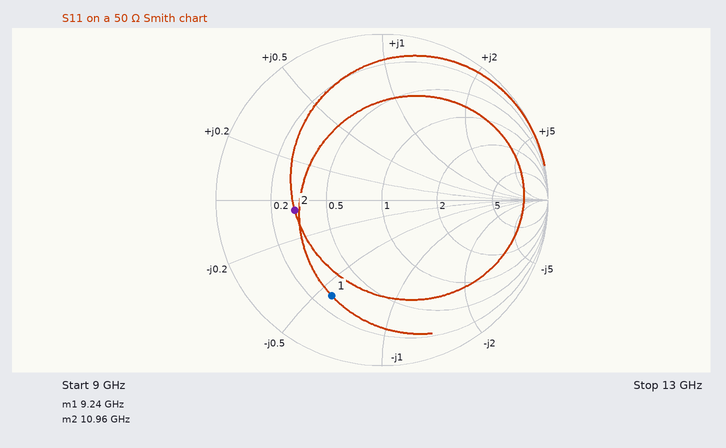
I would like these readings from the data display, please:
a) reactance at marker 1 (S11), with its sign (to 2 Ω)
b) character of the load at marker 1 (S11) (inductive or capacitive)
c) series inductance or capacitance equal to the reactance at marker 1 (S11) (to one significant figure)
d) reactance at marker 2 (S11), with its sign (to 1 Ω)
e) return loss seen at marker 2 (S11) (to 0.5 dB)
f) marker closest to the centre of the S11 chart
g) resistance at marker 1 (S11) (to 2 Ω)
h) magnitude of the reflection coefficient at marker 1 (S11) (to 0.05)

-28 Ω
capacitive
600 fF
-3 Ω
5.5 dB
marker 2
14 Ω
0.65
